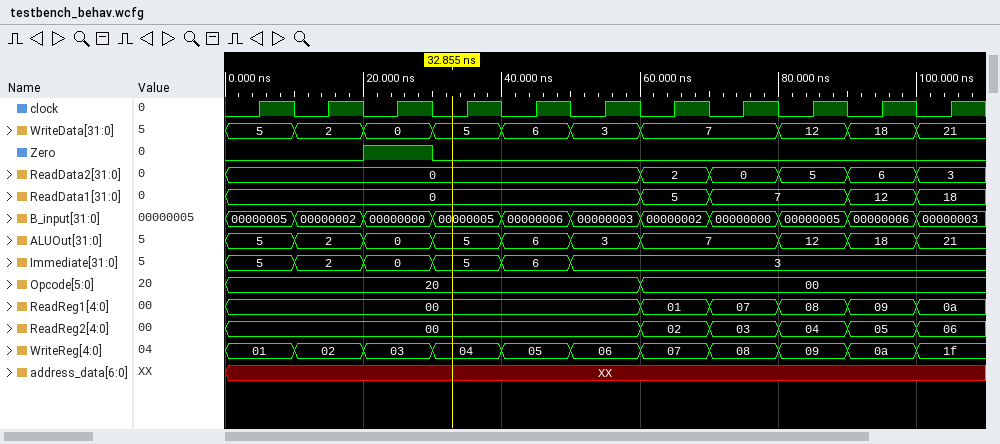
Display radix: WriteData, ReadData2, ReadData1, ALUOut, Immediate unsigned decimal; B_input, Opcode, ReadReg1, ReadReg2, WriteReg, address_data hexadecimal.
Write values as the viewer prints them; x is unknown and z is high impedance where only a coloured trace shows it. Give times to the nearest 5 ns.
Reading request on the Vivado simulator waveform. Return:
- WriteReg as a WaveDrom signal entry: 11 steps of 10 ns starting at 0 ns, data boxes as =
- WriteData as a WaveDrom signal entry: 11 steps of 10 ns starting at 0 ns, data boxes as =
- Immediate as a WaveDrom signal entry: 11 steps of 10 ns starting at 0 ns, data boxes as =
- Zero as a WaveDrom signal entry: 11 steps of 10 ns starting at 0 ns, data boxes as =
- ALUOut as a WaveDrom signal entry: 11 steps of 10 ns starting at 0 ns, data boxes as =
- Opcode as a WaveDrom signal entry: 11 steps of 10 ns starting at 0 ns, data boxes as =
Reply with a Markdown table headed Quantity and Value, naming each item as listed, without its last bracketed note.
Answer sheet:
| Quantity | Value |
|---|---|
| WriteReg as a WaveDrom signal entry: 11 steps of 10 ns starting at 0 ns, data boxes as = | {name: 'WriteReg', wave: '===========', data: '01 02 03 04 05 06 07 08 09 0a 1f'} |
| WriteData as a WaveDrom signal entry: 11 steps of 10 ns starting at 0 ns, data boxes as = | {name: 'WriteData', wave: '=======.===', data: '5 2 0 5 6 3 7 12 18 21'} |
| Immediate as a WaveDrom signal entry: 11 steps of 10 ns starting at 0 ns, data boxes as = | {name: 'Immediate', wave: '======.....', data: '5 2 0 5 6 3'} |
| Zero as a WaveDrom signal entry: 11 steps of 10 ns starting at 0 ns, data boxes as = | {name: 'Zero', wave: '0.10.......'} |
| ALUOut as a WaveDrom signal entry: 11 steps of 10 ns starting at 0 ns, data boxes as = | {name: 'ALUOut', wave: '=======.===', data: '5 2 0 5 6 3 7 12 18 21'} |
| Opcode as a WaveDrom signal entry: 11 steps of 10 ns starting at 0 ns, data boxes as = | {name: 'Opcode', wave: '=.....=....', data: '20 00'} |
